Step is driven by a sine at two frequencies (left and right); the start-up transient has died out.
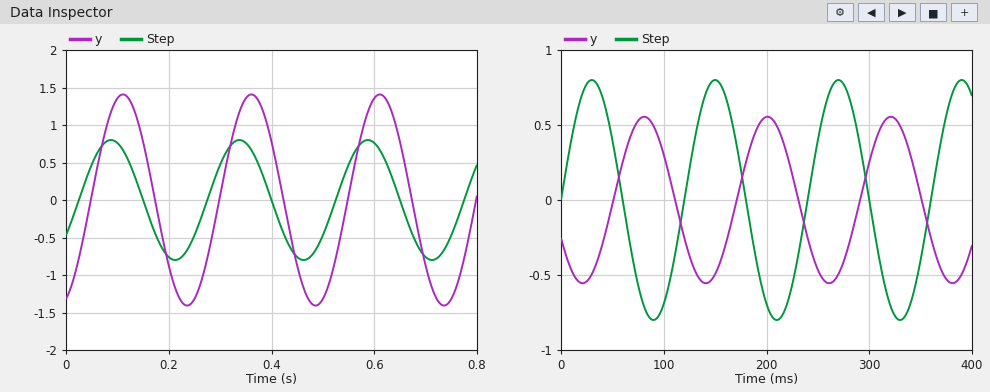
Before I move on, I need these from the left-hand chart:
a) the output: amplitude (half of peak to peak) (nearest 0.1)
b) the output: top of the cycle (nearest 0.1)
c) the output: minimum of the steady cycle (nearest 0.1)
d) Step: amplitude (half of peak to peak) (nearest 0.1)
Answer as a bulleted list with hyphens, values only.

- 1.4
- 1.4
- -1.4
- 0.8
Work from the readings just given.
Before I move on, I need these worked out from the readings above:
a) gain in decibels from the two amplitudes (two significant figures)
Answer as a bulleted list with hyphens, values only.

- 4.9 dB
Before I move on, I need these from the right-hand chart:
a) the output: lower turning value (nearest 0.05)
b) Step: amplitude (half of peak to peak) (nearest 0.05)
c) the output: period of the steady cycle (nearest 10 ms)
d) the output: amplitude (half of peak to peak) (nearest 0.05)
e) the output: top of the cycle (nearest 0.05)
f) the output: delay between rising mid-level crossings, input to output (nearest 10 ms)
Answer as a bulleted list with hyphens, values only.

- -0.55
- 0.80
- 120 ms
- 0.55
- 0.55
- 50 ms
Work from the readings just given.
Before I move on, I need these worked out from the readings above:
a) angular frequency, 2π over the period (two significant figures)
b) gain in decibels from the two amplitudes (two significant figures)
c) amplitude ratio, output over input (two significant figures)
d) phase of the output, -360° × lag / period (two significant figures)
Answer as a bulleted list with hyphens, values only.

- 0.052 rad/ms
- -3.3 dB
- 0.69
- -150°
